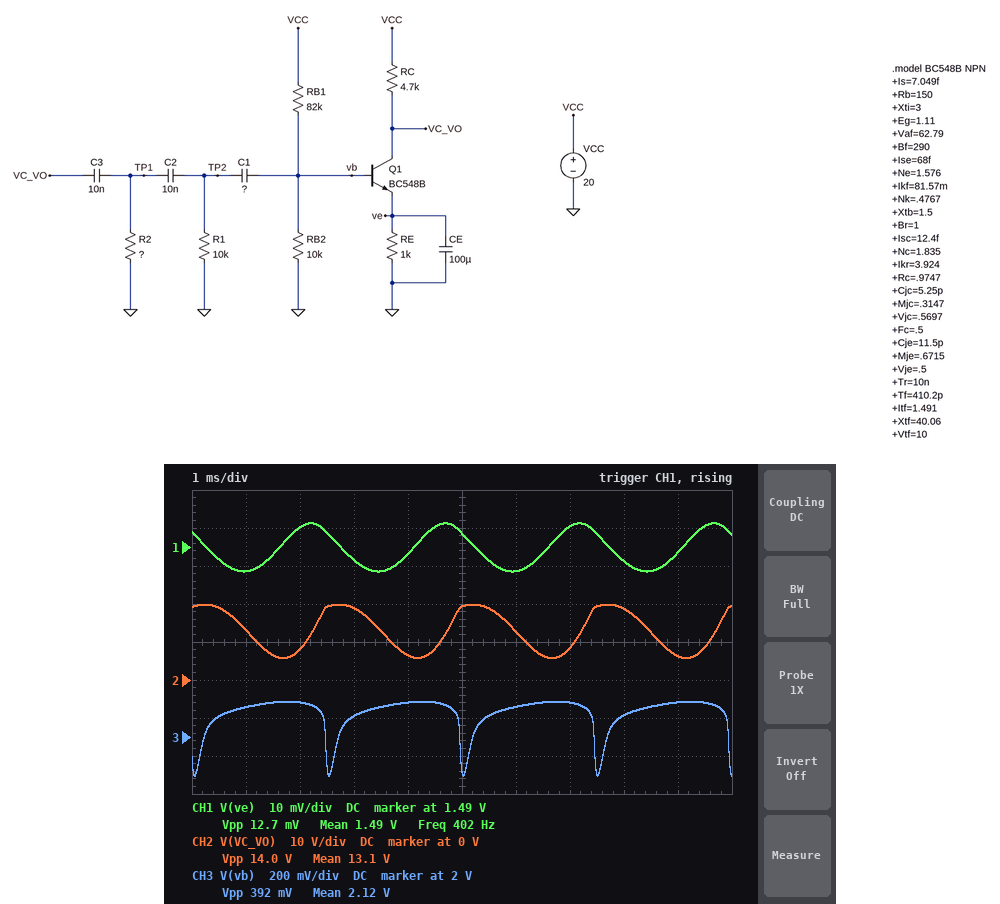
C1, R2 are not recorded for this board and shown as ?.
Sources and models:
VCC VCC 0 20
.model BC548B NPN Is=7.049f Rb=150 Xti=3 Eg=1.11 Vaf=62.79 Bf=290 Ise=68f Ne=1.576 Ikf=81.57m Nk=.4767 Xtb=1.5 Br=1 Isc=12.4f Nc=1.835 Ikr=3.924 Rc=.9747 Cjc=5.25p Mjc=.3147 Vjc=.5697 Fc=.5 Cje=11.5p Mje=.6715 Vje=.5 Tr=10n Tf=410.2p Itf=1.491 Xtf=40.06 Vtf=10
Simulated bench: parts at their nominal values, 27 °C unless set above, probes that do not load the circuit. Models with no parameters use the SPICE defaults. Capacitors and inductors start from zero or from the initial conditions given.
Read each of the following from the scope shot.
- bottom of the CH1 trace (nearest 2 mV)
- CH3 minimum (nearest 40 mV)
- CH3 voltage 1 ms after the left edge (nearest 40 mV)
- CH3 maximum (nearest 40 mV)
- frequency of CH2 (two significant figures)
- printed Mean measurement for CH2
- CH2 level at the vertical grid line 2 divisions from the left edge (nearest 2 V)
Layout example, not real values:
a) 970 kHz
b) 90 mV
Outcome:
a) 1.484 V
b) 1.80 V
c) 2.16 V
d) 2.20 V
e) 400 Hz
f) 13.1 V
g) 8 V
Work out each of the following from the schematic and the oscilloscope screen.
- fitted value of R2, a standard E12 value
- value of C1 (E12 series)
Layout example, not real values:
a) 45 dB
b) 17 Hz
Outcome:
a) 12 kΩ
b) 18 nF
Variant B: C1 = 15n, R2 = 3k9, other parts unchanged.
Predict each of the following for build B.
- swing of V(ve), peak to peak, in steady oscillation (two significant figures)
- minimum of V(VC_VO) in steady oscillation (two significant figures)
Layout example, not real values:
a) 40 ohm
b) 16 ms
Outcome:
a) 8.0 mV
b) 6.0 V
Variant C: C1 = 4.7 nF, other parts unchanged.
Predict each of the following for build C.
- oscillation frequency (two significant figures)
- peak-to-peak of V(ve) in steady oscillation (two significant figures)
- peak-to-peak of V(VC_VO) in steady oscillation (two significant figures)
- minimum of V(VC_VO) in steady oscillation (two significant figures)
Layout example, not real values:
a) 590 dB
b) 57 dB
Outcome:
a) 640 Hz
b) 7.7 mV
c) 13 V
d) 6.3 V
